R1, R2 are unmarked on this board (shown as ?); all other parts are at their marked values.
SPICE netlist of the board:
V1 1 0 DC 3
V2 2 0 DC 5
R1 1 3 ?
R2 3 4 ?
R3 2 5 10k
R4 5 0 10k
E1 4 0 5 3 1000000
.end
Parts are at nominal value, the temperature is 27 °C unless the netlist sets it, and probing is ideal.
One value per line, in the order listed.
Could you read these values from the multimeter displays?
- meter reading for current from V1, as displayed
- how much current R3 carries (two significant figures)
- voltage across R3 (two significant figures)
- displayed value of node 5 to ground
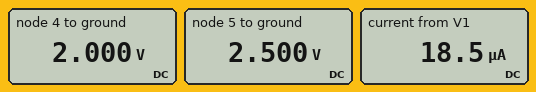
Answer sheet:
18.5 µA
250 µA
2.5 V
2.500 V
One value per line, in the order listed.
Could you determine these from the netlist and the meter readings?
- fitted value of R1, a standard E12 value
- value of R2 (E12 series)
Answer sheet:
27 kΩ
27 kΩ
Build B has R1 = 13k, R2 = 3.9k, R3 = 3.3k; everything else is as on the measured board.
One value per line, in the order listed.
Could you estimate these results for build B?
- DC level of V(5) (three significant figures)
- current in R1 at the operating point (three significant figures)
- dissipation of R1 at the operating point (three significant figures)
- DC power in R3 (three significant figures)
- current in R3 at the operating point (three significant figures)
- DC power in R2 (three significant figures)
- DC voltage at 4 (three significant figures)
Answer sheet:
3.76 V
58.4 µA
44.4 µW
466 µW
376 µA
13.3 µW
3.99 V
